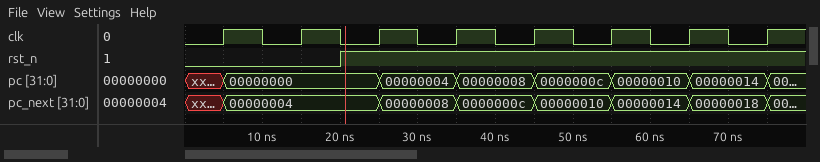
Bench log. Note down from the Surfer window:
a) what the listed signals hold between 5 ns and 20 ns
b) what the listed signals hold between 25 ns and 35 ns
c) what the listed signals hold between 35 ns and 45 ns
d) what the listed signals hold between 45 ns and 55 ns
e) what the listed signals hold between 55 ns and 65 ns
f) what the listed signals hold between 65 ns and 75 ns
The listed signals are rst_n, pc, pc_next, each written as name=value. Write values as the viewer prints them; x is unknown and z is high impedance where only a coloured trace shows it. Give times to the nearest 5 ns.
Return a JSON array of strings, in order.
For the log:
["rst_n=0, pc=00000000, pc_next=00000004", "rst_n=1, pc=00000004, pc_next=00000008", "rst_n=1, pc=00000008, pc_next=0000000c", "rst_n=1, pc=0000000c, pc_next=00000010", "rst_n=1, pc=00000010, pc_next=00000014", "rst_n=1, pc=00000014, pc_next=00000018"]
